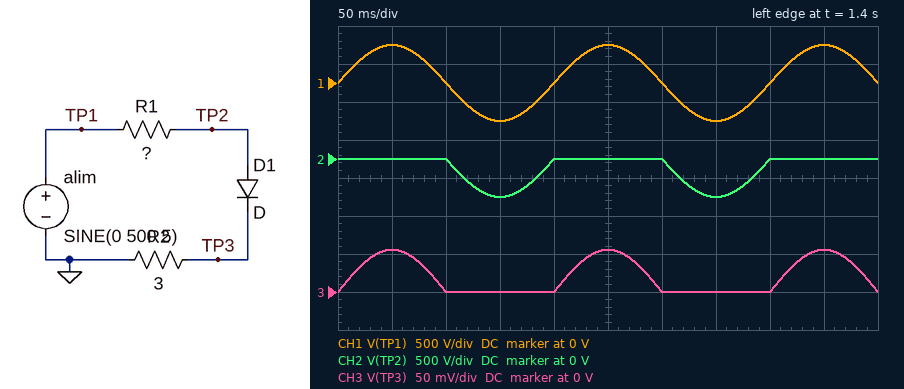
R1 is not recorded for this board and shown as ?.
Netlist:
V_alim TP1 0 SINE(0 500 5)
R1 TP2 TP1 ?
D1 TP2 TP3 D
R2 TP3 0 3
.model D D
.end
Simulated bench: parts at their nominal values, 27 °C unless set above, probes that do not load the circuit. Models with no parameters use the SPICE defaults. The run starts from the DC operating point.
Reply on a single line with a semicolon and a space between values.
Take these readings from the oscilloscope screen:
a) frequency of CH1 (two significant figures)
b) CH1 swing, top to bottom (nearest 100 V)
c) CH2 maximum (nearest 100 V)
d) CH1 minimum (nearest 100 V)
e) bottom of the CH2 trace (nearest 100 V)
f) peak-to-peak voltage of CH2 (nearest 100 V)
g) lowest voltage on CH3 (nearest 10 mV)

5.0 Hz; 1.0 kV; 0 V; -500 V; -500 V; 500 V; 0 V
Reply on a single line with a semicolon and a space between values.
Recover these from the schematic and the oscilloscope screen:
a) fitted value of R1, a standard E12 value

27 kΩ
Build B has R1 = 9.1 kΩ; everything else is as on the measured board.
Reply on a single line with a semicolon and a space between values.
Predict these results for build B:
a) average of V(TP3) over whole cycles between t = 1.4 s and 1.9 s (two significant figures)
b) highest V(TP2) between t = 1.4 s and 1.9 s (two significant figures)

52 mV; 920 mV
